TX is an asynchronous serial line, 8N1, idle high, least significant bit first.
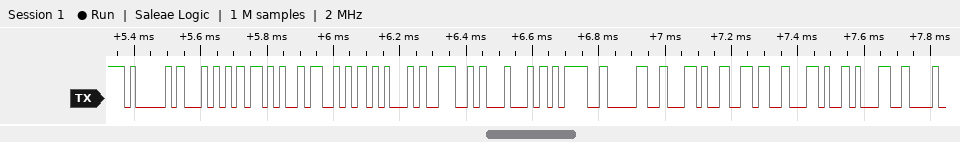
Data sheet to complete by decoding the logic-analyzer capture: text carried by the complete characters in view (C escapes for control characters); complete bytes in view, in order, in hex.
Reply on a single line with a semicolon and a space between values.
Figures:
"AT+SEND=0,6,1"; 41 54 2B 53 45 4E 44 3D 30 2C 36 2C 31
